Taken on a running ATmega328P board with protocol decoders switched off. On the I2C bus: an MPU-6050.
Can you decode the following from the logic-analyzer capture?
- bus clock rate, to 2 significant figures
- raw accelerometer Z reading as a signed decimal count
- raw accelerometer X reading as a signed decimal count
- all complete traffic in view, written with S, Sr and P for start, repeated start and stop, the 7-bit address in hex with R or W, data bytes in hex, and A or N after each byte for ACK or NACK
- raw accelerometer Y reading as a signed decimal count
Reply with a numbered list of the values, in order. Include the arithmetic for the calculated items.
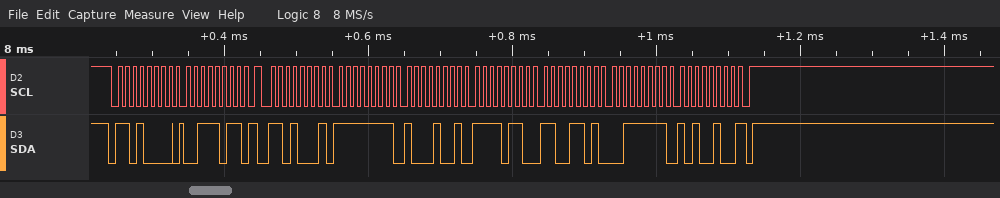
1. 100 kHz
2. 0x3FA4 = 16292
3. 0xFF89 = -119
4. S 68W A 3B A Sr 68R A FF A 89 A F6 A CD A 3F A A4 N P
5. 0xF6CD = -2355
